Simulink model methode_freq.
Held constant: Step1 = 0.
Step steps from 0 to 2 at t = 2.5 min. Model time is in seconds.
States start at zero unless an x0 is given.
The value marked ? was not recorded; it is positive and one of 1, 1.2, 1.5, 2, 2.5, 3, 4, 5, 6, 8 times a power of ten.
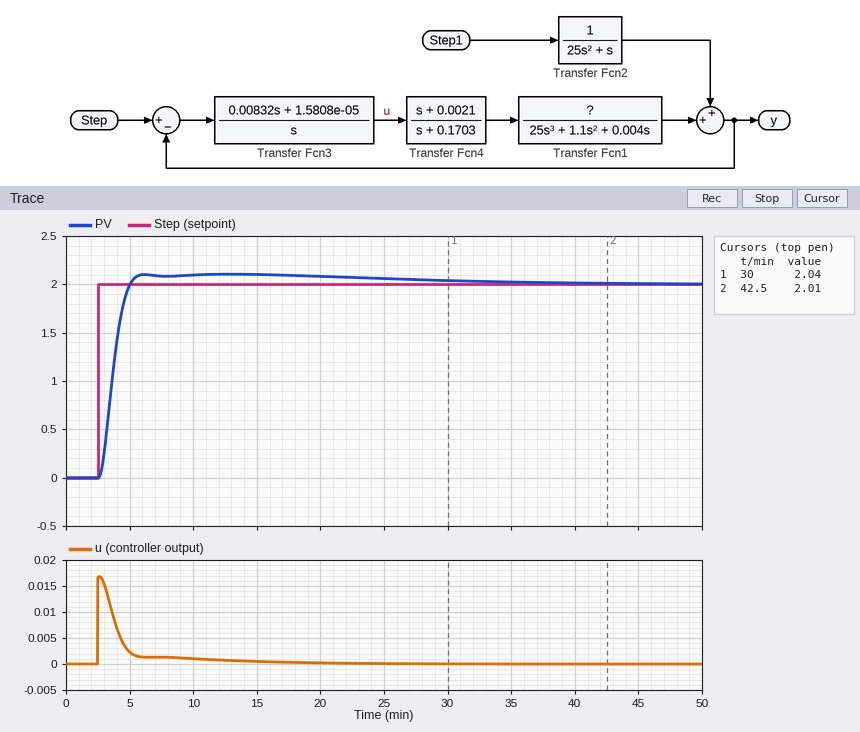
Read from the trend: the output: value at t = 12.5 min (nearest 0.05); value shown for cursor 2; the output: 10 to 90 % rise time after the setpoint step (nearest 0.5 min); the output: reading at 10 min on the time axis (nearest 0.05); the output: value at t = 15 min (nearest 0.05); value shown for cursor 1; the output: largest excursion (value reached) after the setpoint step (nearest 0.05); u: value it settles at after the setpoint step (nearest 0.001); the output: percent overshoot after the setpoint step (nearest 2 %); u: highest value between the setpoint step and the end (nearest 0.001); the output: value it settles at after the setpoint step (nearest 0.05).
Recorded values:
2.10
2.01
1.5 min
2.10
2.10
2.04
2.10
0.000
6 %
0.017
2.00
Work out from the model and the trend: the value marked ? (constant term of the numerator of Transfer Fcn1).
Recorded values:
0.3
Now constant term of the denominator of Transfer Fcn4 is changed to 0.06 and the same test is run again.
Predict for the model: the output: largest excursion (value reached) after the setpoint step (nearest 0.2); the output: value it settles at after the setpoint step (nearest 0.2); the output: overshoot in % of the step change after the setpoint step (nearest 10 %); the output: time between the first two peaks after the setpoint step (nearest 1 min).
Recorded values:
3.0
2.0
50 %
3 min
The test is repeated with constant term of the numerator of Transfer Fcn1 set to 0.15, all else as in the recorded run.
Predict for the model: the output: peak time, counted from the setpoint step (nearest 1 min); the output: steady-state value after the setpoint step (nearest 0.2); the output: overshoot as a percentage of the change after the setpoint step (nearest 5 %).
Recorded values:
14 min
2.0
10 %
